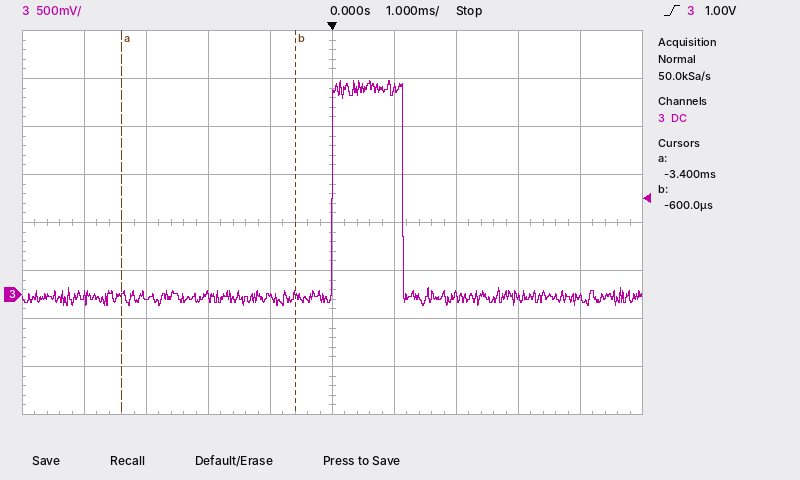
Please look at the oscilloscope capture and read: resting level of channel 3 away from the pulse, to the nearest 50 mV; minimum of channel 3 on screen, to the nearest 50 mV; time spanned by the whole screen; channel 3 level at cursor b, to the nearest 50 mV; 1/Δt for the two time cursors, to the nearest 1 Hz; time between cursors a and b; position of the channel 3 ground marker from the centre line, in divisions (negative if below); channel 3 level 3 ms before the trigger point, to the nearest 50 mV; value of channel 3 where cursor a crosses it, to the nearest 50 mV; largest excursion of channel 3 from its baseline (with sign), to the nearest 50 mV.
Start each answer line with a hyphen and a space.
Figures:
- -50 mV
- -100 mV
- 10 ms
- 0 mV
- 357 Hz
- 2.8 ms
- -1.5 div
- 0 mV
- 0 mV
- +2.25 V
